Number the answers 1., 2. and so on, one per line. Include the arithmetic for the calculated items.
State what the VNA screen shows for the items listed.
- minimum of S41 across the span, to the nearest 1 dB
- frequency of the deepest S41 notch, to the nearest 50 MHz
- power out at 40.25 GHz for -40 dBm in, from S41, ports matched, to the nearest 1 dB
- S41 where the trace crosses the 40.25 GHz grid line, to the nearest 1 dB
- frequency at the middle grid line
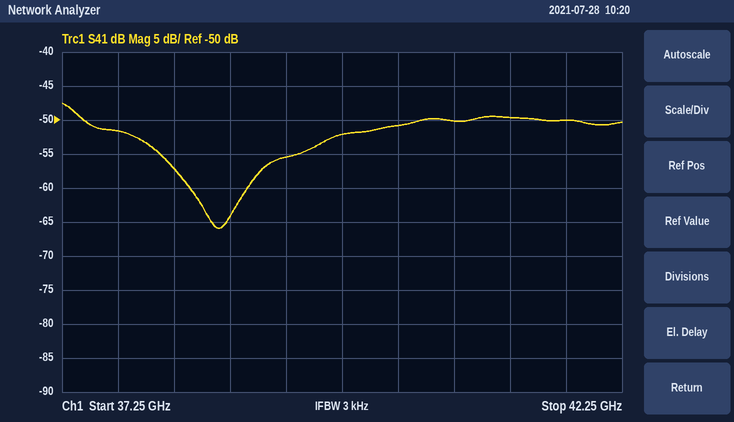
1. -66 dB
2. 38.65 GHz
3. -40 dBm + (-51 dB) = -91 dBm
4. -51 dB
5. 39.75 GHz
